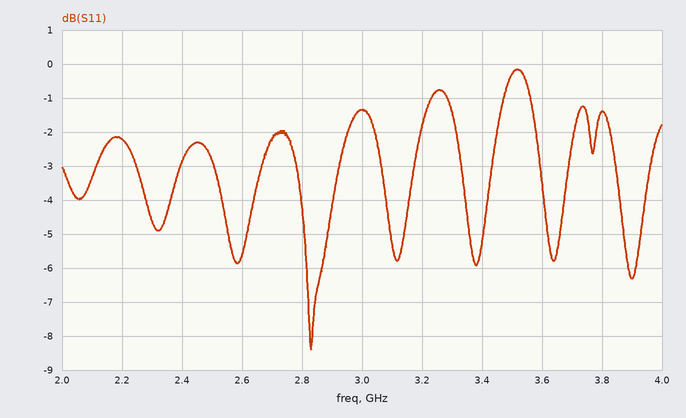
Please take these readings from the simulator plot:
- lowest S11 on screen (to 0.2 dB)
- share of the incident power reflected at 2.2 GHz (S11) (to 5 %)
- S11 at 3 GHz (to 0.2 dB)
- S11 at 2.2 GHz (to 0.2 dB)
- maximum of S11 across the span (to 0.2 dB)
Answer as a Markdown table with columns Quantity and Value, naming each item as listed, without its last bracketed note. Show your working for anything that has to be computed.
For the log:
| Quantity | Value |
|---|---|
| lowest S11 on screen | -8.4 dB |
| share of the incident power reflected at 2.2 GHz (S11) | 10^(-2.2/10) ≈ 60 % |
| S11 at 3 GHz | -1.4 dB |
| S11 at 2.2 GHz | -2.2 dB |
| maximum of S11 across the span | -0.2 dB |
